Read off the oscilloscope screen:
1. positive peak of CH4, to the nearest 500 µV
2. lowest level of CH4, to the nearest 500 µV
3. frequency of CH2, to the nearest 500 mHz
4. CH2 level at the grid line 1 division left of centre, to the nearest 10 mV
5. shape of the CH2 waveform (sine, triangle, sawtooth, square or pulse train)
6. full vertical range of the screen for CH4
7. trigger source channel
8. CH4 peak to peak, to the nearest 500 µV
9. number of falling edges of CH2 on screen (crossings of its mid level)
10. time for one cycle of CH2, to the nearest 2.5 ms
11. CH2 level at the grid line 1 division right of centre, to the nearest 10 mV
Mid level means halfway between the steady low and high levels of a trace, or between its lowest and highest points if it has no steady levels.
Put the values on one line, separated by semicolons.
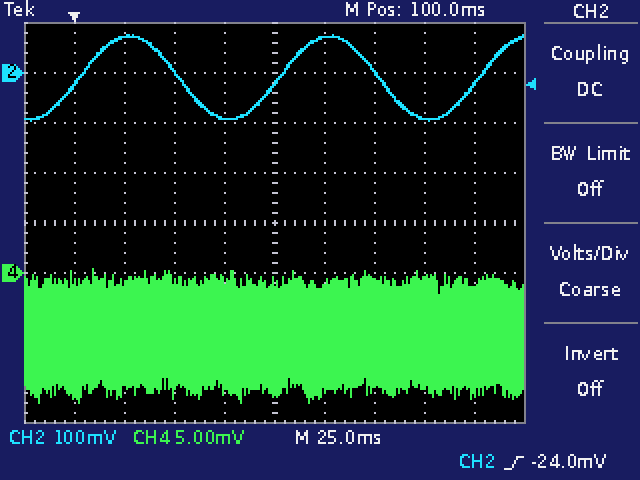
500 µV; -13.0 mV; 10.0 Hz; -90 mV; sine; 40 mV; CH2; 13.5 mV; 2; 100.0 ms; 70 mV
